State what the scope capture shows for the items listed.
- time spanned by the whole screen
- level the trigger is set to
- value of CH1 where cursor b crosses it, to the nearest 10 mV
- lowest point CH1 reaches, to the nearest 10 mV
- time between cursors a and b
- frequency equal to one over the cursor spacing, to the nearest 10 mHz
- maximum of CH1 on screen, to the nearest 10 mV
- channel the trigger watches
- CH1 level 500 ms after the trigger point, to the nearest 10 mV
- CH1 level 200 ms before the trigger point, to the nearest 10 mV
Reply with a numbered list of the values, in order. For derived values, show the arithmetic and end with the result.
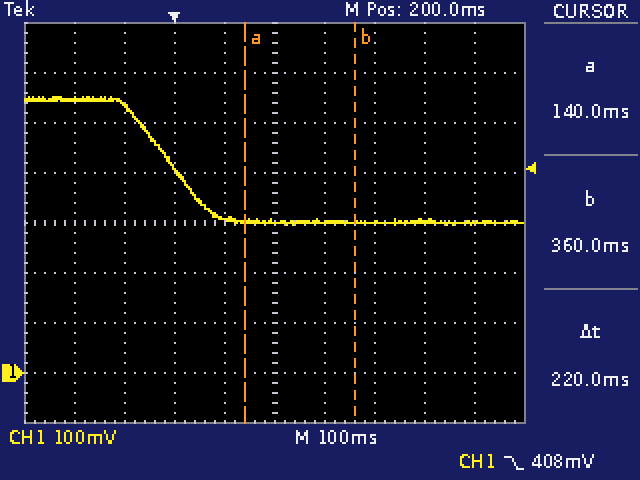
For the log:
1. 1 s
2. 408 mV
3. 300 mV
4. 300 mV
5. 220 ms
6. 1 / 220 ms ≈ 4.55 Hz
7. 550 mV
8. CH1
9. 300 mV
10. 550 mV
